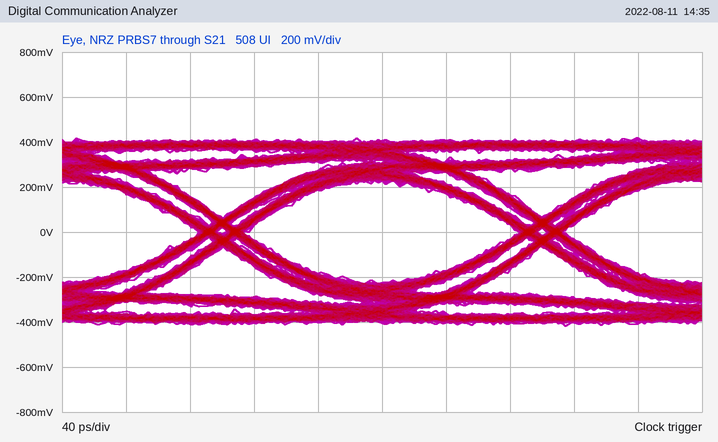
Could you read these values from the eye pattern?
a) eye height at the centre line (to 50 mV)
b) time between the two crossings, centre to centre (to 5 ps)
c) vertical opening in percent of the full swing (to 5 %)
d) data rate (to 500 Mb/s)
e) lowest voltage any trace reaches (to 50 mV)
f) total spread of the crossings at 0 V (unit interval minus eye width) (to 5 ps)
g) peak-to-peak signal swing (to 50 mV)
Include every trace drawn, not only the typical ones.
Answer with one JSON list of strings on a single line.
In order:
["450 mV", "200 ps", "55 %", "5.0 Gb/s", "-400 mV", "30 ps", "850 mV"]
